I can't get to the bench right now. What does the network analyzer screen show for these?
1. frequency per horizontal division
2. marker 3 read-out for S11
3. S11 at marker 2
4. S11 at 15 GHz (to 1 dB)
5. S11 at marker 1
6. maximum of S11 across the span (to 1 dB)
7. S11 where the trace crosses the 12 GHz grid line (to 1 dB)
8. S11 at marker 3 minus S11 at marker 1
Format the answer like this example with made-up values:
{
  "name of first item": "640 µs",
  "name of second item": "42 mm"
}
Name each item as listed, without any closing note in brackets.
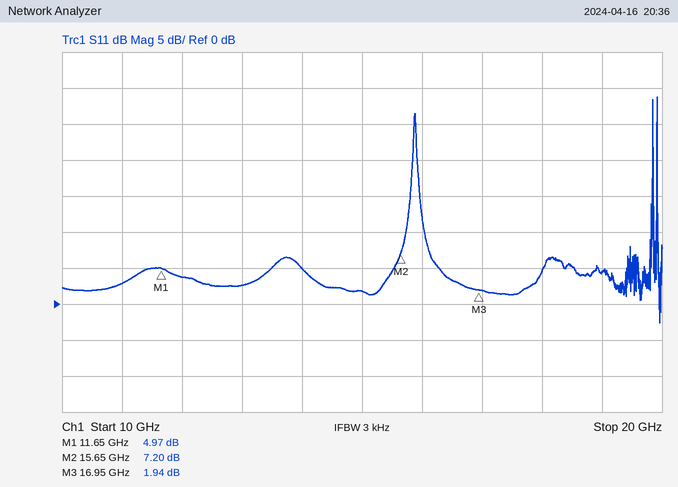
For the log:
{
  "frequency per horizontal division": "1 GHz",
  "marker 3 read-out for S11": "1.94 dB",
  "S11 at marker 2": "7.20 dB",
  "S11 at 15 GHz": "2 dB",
  "S11 at marker 1": "4.97 dB",
  "maximum of S11 across the span": "29 dB",
  "S11 where the trace crosses the 12 GHz grid line": "4 dB",
  "S11 at marker 3 minus S11 at marker 1": "-3.03 dB"
}
